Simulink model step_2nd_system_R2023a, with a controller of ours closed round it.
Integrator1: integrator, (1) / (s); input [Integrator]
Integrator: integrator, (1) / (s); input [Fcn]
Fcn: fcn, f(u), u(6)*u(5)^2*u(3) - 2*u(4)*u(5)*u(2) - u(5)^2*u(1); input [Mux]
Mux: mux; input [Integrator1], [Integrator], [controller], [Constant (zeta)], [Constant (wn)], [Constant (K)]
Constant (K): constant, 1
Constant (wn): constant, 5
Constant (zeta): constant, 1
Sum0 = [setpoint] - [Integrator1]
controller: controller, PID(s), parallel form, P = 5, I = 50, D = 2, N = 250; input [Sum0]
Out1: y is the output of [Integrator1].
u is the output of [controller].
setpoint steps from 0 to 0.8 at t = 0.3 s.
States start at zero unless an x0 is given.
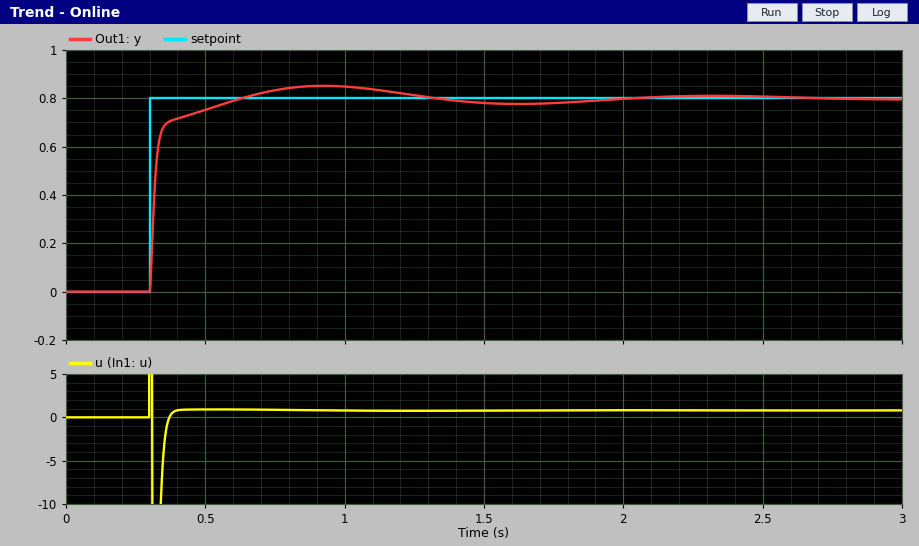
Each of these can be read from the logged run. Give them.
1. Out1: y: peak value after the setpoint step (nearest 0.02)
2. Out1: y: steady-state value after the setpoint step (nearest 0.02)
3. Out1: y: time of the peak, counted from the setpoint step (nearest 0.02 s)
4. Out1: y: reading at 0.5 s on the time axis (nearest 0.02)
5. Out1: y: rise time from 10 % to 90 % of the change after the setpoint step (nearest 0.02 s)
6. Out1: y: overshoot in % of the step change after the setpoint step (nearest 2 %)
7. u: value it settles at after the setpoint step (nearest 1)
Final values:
0.86
0.80
0.62 s
0.76
0.10 s
6 %
1
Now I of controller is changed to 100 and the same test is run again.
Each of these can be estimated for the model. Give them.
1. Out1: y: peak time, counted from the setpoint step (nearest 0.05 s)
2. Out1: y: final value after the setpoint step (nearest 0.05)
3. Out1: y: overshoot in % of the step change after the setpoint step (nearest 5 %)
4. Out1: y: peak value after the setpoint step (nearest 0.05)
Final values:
0.40 s
0.80
10 %
0.90
